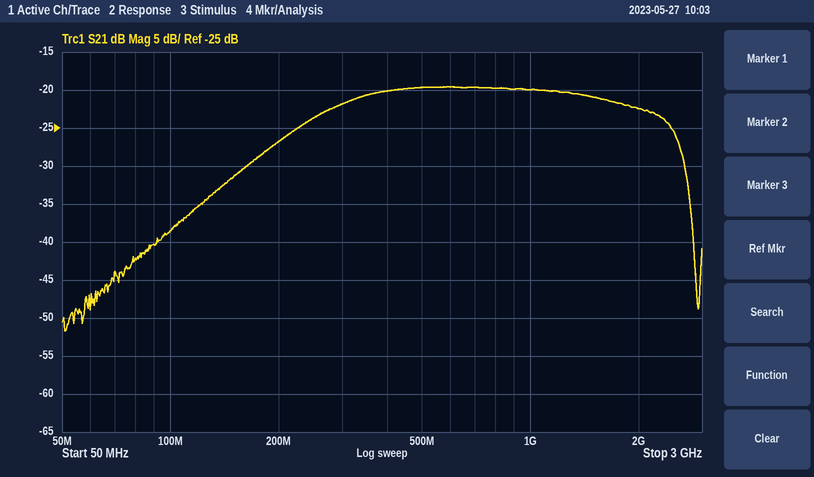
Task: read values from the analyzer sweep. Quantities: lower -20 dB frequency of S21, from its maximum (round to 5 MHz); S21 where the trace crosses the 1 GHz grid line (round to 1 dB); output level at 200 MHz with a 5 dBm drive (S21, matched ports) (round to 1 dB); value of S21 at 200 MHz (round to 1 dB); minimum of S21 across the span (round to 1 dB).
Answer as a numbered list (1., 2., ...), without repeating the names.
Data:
1. 95 MHz
2. -20 dB
3. -22 dBm
4. -27 dB
5. -52 dB
